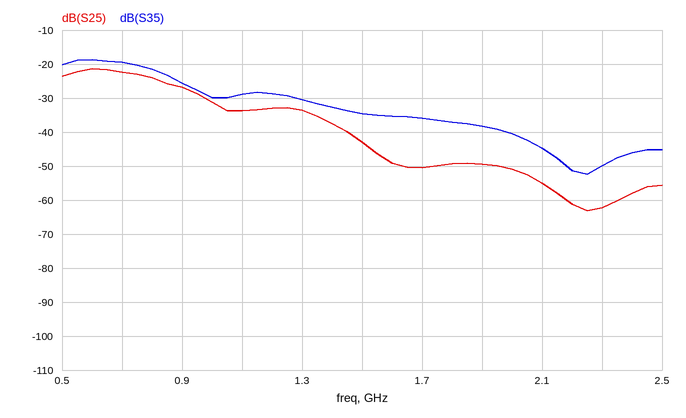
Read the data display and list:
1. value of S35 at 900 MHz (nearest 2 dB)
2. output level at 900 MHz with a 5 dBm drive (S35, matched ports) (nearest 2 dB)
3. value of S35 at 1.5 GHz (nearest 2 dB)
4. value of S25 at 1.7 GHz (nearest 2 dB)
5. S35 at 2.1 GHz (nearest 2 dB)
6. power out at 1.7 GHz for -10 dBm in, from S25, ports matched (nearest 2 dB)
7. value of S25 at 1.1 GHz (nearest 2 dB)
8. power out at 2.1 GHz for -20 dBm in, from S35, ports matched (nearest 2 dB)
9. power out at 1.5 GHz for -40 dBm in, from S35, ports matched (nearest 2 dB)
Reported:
-26 dB
-20 dBm
-34 dB
-50 dB
-44 dB
-60 dBm
-34 dB
-64 dBm
-74 dBm
